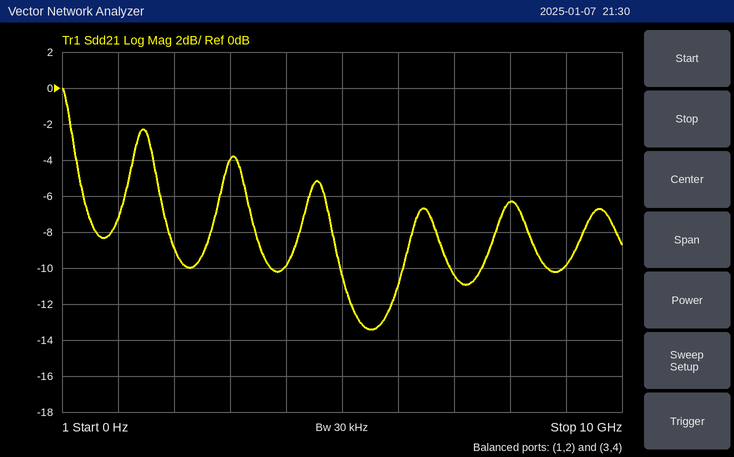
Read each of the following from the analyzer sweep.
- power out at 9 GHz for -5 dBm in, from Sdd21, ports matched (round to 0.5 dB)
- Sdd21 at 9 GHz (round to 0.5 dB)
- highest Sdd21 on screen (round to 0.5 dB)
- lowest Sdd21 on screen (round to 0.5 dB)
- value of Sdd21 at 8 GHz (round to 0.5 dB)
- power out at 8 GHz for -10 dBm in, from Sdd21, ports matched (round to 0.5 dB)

-15.0 dBm
-10.0 dB
0.0 dB
-13.5 dB
-6.5 dB
-16.5 dBm
